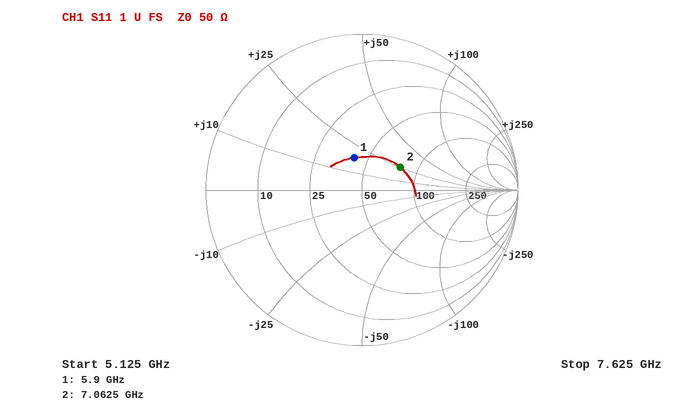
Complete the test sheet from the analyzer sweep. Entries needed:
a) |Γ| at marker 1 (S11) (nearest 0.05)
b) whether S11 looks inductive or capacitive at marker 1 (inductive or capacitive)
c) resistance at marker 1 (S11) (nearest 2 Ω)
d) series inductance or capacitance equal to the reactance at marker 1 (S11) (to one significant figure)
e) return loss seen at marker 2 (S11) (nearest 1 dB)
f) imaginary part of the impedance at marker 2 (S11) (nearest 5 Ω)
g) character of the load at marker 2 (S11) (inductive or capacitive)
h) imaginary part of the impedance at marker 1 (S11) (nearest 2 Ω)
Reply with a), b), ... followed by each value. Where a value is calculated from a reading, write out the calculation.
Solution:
a) 0.20
b) inductive
c) 42 Ω
d) L = 18 Ω/(2π × 5.9 GHz) ≈ 486 pH, so 500 pH to one significant figure
e) 11 dB
f) +25 Ω
g) inductive
h) +18 Ω
